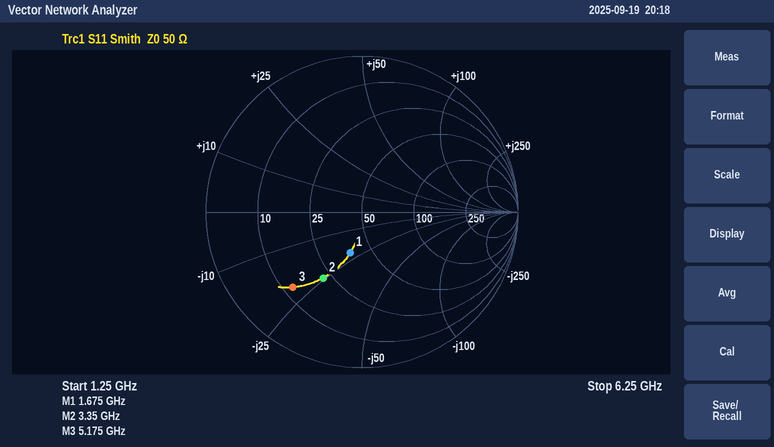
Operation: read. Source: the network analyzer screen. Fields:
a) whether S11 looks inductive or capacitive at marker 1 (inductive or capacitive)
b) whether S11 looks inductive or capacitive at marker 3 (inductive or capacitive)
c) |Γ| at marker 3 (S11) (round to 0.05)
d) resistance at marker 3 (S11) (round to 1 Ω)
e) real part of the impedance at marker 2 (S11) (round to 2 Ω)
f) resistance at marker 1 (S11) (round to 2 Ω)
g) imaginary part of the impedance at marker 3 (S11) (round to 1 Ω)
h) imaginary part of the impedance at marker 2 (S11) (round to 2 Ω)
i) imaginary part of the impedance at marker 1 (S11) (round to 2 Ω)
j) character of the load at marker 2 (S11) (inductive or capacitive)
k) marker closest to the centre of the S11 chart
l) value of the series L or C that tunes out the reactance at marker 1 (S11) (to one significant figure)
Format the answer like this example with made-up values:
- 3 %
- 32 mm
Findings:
- capacitive
- capacitive
- 0.65
- 12 Ω
- 22 Ω
- 38 Ω
- -21 Ω
- -24 Ω
- -22 Ω
- capacitive
- marker 1
- 2 nH
